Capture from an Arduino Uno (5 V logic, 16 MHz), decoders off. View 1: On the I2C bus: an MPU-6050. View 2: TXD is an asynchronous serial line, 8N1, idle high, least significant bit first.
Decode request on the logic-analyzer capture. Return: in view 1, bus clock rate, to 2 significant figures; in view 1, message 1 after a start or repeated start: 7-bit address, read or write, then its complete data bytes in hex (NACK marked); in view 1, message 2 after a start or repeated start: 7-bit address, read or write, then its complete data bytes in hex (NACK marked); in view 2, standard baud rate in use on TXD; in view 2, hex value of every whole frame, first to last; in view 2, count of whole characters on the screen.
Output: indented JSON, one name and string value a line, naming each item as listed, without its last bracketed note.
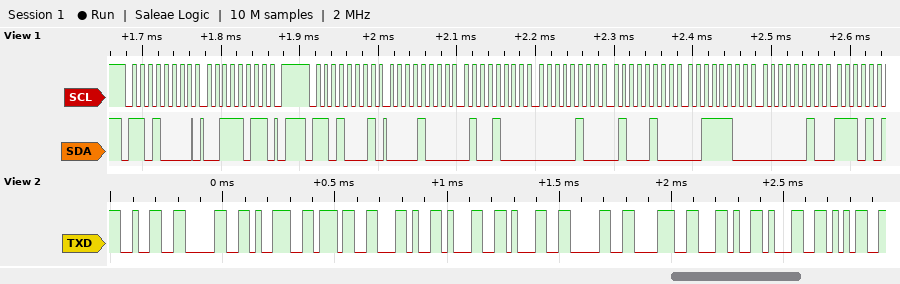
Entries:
{
  "in view 1, bus clock rate, to 2 significant figures": "100 kHz",
  "in view 1, message 1 after a start or repeated start: 7-bit address, read or write, then its complete data bytes in hex": "0x68 write: 3B",
  "in view 1, message 2 after a start or repeated start: 7-bit address, read or write, then its complete data bytes in hex": "0x68 read: 08 48 04 44 3C 02",
  "in view 2, standard baud rate in use on TXD": "38400 baud",
  "in view 2, hex value of every whole frame, first to last": "32 30 39 37 2C 31 31 30 38 2C 31 35",
  "in view 2, count of whole characters on the screen": "12"
}
